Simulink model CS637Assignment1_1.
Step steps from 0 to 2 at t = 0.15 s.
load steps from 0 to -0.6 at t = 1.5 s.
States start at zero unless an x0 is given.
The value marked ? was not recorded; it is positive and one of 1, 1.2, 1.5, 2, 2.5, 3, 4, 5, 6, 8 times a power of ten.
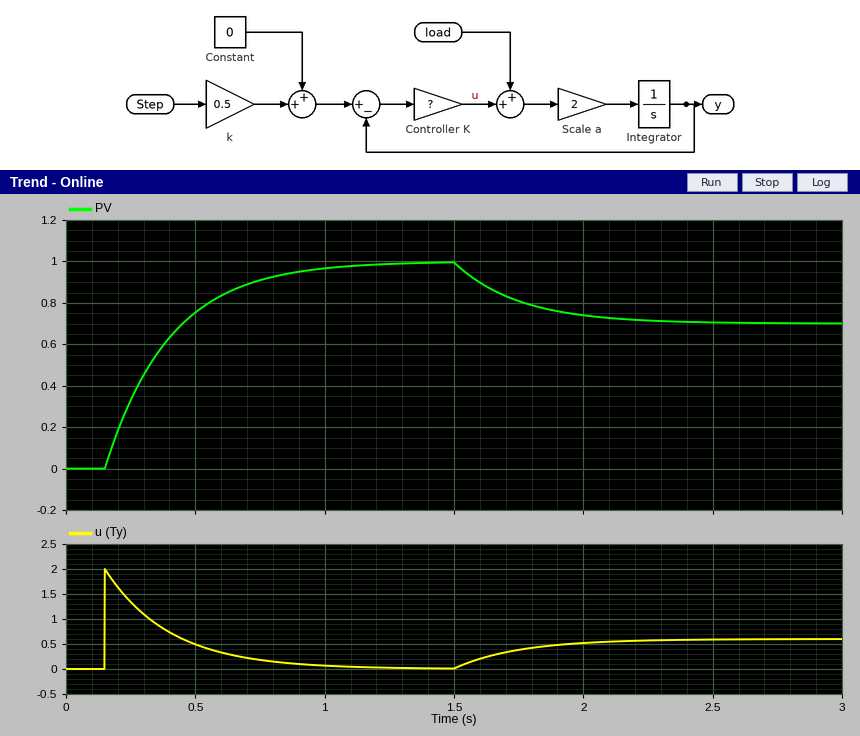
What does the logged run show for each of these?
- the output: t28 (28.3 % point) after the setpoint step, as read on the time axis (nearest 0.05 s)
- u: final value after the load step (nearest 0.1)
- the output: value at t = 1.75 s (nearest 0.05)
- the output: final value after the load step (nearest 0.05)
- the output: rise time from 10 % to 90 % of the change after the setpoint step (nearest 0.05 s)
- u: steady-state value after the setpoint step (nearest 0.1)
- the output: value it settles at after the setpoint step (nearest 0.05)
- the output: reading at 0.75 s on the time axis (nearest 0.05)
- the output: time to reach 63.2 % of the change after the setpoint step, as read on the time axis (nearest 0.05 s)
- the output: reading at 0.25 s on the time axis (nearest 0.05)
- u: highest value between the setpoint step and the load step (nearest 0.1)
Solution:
0.25 s
0.6
0.80
0.70
0.55 s
0.0
1.00
0.90
0.40 s
0.35
2.0
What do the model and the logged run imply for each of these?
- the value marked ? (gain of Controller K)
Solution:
2
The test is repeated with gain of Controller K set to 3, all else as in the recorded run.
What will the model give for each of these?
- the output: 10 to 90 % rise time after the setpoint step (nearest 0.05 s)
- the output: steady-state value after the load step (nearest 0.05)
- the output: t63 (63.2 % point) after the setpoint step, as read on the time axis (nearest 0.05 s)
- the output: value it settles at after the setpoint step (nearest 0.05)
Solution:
0.35 s
0.80
0.30 s
1.00
